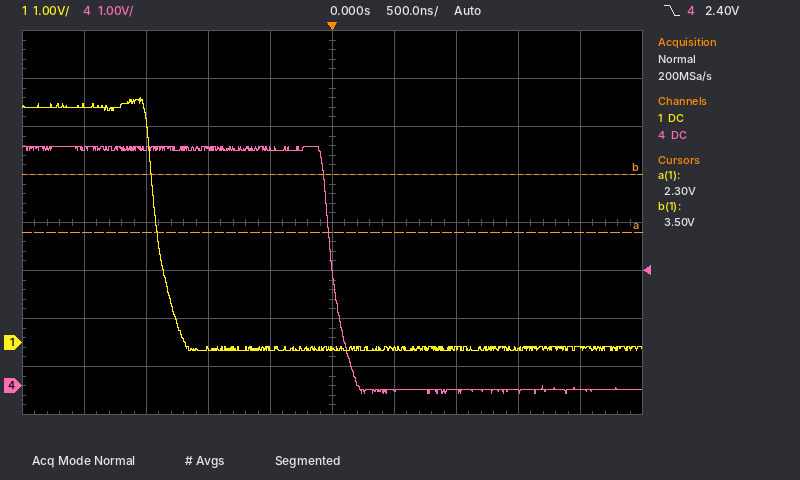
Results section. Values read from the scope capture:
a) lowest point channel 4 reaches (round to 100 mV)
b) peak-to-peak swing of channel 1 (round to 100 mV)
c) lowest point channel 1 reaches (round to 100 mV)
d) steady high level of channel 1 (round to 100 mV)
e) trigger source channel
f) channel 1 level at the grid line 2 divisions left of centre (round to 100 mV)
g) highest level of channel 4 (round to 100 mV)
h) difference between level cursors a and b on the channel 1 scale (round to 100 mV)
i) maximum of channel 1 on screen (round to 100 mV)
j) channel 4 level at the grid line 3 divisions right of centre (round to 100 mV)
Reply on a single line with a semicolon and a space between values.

-200 mV; 5.3 V; -200 mV; 4.9 V; channel 4; -100 mV; 5.0 V; 1.2 V; 5.1 V; -100 mV
